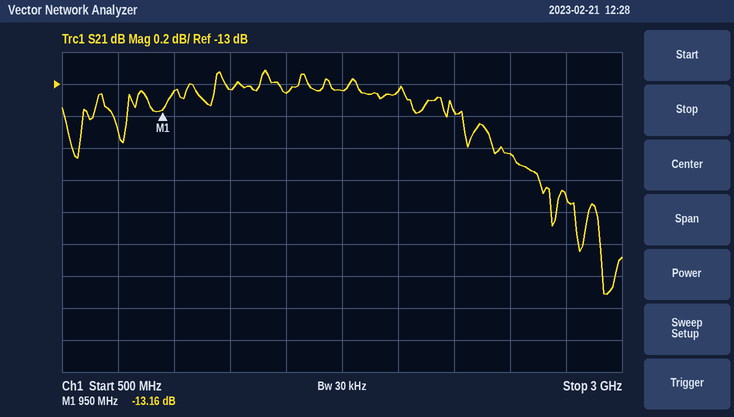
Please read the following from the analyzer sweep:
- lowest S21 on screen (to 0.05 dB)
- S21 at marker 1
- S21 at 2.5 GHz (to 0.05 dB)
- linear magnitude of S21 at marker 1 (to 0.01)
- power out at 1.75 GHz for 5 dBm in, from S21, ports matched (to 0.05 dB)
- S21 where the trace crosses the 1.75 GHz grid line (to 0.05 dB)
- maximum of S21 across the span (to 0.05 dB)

-14.30 dB
-13.16 dB
-13.45 dB
0.22
-8.05 dBm
-13.05 dB
-12.90 dB
